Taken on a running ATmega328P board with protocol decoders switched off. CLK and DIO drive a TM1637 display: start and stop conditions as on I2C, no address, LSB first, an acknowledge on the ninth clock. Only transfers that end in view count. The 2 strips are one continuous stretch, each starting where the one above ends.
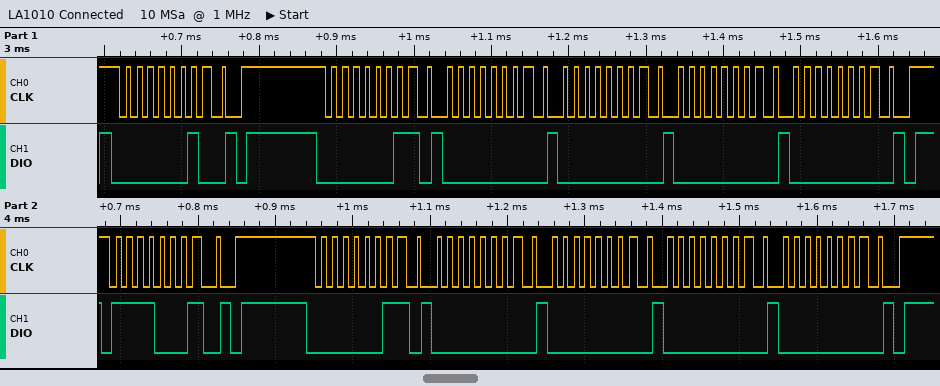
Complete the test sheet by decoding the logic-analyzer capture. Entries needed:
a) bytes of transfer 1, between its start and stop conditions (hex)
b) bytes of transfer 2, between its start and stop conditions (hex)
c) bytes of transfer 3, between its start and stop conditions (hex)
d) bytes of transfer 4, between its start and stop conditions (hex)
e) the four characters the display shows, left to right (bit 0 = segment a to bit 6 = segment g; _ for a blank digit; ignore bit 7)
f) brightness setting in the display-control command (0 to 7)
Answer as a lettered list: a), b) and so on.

a) 40
b) C0 00 00 00 00
c) 8F
d) C0 00 00 00 00
e) ____
f) 7
